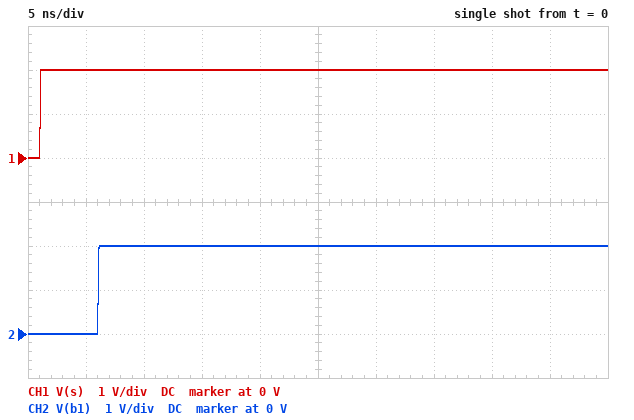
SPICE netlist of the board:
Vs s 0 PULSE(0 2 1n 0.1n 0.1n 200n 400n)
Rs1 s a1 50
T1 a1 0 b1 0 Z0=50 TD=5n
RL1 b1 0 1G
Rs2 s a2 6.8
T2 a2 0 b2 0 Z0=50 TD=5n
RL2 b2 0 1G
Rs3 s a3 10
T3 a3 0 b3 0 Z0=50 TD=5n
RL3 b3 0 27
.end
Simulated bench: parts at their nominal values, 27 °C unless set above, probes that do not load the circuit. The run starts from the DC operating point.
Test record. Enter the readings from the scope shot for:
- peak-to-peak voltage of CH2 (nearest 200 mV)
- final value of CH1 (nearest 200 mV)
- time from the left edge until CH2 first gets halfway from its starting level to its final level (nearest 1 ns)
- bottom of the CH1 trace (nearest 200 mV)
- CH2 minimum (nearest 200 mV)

2.0 V
2.0 V
6 ns
0 V
0 V
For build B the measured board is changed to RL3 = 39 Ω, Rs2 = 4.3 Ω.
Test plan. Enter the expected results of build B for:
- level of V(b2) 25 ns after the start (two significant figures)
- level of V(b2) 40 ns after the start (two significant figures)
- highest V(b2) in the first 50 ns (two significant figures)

580 mV
1.0 V
3.7 V
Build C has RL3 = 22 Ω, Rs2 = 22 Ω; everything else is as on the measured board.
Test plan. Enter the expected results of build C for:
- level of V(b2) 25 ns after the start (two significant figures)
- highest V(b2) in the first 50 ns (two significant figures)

1.7 V
2.8 V
